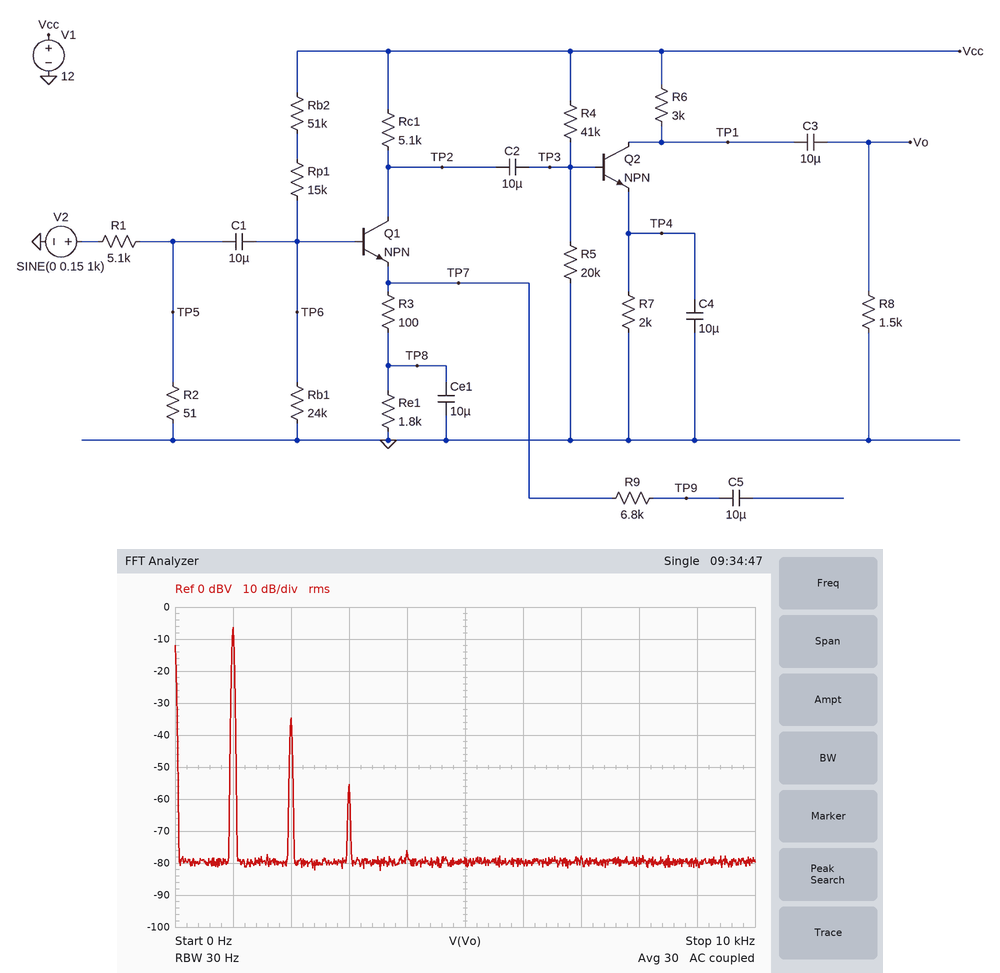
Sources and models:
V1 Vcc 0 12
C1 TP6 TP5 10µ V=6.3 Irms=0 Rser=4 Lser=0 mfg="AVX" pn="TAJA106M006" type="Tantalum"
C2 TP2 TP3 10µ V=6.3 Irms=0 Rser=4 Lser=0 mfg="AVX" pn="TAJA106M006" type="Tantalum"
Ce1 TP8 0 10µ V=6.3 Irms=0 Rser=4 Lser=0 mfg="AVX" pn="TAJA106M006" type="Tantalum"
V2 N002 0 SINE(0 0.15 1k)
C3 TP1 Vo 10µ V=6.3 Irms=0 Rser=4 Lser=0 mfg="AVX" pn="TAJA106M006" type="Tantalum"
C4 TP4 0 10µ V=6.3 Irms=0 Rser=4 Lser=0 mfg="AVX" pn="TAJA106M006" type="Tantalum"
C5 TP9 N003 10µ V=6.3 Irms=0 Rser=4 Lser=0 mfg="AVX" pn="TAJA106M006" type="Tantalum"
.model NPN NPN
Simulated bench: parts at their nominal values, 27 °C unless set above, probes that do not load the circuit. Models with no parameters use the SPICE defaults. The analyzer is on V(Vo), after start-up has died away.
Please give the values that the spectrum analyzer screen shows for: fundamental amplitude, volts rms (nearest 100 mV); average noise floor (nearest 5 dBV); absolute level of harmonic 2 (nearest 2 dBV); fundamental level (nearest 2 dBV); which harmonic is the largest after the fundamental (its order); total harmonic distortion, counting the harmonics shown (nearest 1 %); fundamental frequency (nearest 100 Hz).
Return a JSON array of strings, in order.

["500 mV", "-80 dBV", "-34 dBV", "-6 dBV", "2", "4 %", "1.0 kHz"]
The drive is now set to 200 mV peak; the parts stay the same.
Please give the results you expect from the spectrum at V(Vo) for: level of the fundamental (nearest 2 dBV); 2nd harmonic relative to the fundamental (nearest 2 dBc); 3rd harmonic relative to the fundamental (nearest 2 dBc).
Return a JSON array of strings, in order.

["-4 dBV", "-26 dBc", "-44 dBc"]
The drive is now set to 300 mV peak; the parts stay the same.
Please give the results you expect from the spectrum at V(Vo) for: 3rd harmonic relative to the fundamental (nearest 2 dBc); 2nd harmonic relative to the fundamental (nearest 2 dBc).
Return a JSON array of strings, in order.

["-36 dBc", "-20 dBc"]
